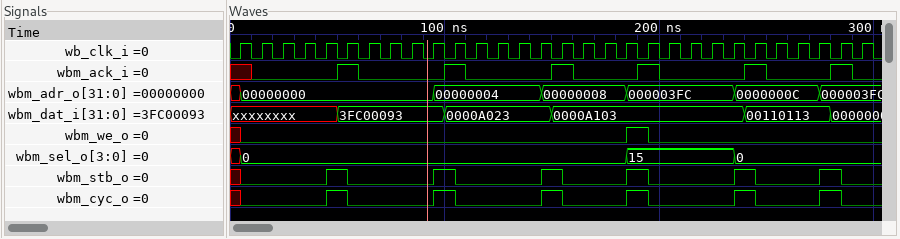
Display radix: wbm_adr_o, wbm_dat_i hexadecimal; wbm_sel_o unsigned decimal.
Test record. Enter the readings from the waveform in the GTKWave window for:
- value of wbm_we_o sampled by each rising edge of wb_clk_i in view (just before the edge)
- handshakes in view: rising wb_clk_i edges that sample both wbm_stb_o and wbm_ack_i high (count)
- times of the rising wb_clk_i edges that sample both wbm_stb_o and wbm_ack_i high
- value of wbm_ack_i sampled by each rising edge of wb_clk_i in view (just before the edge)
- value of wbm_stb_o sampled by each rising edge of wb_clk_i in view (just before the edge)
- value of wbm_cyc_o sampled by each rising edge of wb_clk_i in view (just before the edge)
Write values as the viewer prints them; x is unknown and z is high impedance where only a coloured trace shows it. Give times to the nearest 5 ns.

x 0 0 0 0 0 0 0 0 0 0 0 0 0 0 0 0 0 0 1 0 0 0 0 0 0 0 0 0 0
6
55 ns, 105 ns, 155 ns, 195 ns, 245 ns, 285 ns
x 0 0 0 0 1 0 0 0 0 1 0 0 0 0 1 0 0 0 1 0 0 0 0 1 0 0 0 1 0
x 0 0 0 0 1 0 0 0 0 1 0 0 0 0 1 0 0 0 1 0 0 0 0 1 0 0 0 1 0
x 0 0 0 0 1 0 0 0 0 1 0 0 0 0 1 0 0 0 1 0 0 0 0 1 0 0 0 1 0
